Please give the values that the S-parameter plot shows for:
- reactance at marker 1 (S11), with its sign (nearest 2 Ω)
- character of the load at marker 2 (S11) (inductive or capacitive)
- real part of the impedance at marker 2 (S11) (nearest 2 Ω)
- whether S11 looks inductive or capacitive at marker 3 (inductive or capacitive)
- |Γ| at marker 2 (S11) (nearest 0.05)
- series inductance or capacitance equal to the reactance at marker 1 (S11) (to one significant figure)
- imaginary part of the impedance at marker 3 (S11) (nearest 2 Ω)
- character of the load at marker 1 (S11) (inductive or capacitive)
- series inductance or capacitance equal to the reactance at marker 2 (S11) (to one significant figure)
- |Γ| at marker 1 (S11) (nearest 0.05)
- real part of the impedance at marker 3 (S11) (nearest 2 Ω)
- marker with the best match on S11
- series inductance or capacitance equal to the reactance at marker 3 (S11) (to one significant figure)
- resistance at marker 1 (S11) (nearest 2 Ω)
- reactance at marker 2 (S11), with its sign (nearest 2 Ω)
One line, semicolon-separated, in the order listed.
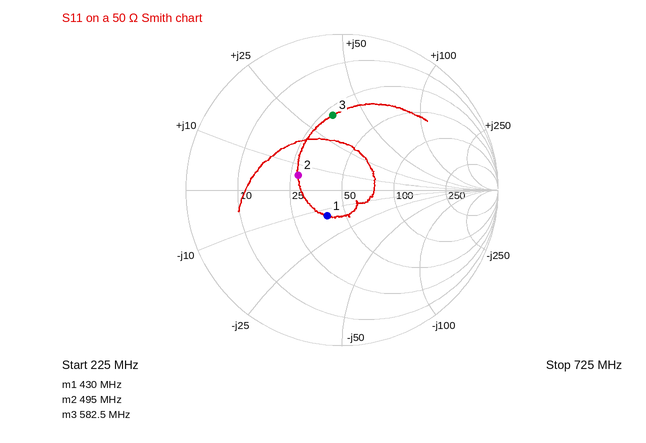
-14 Ω; inductive; 28 Ω; inductive; 0.30; 30 pF; +36 Ω; capacitive; 2 nH; 0.20; 28 Ω; marker 1; 10 nH; 40 Ω; +6 Ω
